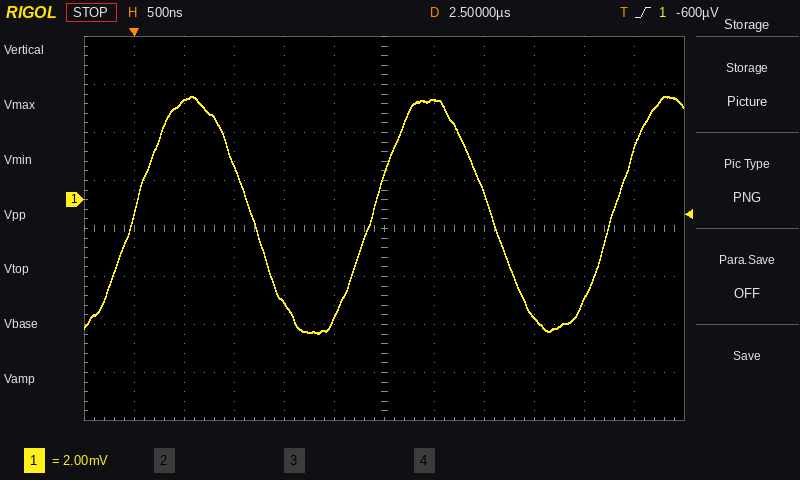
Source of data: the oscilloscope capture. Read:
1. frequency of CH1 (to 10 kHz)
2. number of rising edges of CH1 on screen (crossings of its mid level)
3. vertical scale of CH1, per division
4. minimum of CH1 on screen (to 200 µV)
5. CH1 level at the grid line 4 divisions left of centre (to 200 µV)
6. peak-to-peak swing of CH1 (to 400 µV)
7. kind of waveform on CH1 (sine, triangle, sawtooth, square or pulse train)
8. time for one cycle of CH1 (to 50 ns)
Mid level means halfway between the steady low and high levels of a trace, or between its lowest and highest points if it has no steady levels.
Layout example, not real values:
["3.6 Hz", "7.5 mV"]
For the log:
["420 kHz", "3", "2 mV", "-5.6 mV", "4.2 mV", "10.0 mV", "sine", "2.40 µs"]
